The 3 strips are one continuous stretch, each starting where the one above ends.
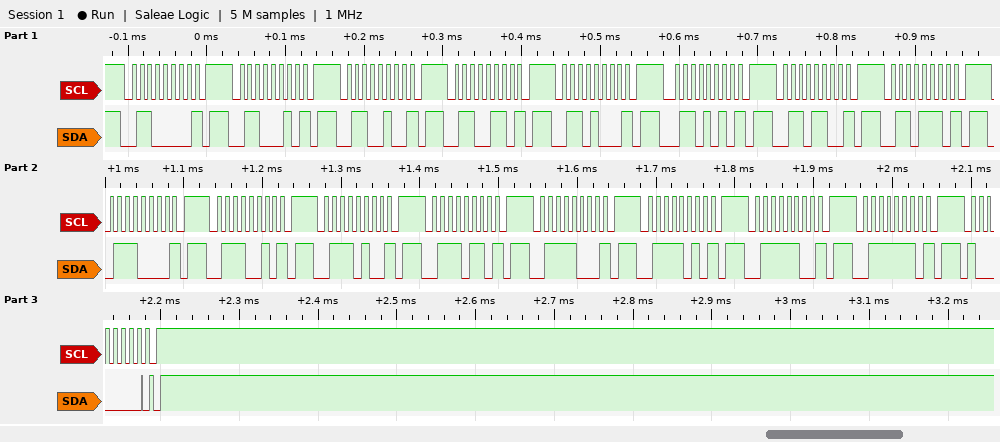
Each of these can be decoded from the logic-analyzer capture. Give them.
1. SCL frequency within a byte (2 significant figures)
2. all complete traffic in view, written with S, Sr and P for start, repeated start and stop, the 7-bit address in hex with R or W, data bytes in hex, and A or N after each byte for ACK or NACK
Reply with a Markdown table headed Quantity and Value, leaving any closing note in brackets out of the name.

| Quantity | Value |
|---|---|
| SCL frequency within a byte | 100 kHz |
| all complete traffic in view, written with S, Sr and P for start, repeated start and stop, the 7-bit address in hex with R or W, data bytes in hex, and A or N after each byte for ACK or NACK | S 30W N P S 31W N P S 32W N P S 33W N P S 34W N P S 35W N P S 36W N P S 37W N P S 38W N P S 39W N P S 3AW N P S 3BW N P S 3CW N P S 3DW N P S 3EW N P S 3FW N P S 40W A P |
